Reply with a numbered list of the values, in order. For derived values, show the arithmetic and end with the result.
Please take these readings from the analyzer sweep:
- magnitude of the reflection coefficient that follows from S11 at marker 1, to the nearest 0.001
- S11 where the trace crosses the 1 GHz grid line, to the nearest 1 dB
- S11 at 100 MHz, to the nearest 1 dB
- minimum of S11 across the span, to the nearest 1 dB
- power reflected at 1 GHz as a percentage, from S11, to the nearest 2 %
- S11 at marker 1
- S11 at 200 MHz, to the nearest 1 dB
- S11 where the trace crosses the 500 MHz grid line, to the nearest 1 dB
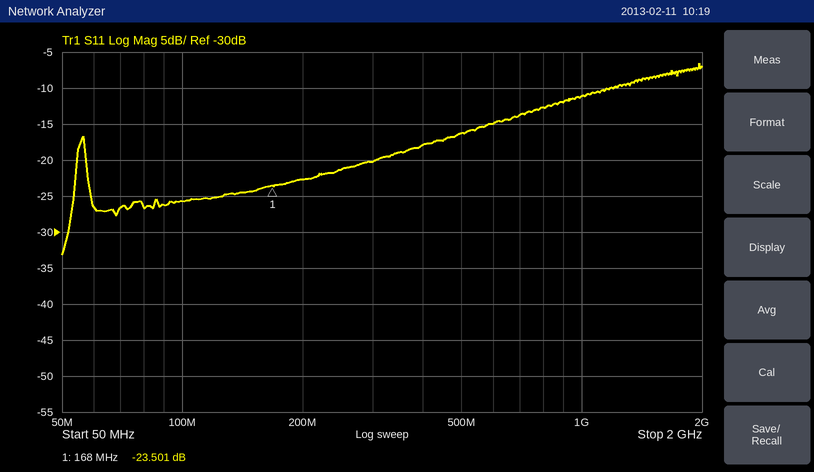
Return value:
1. 10^(-23.501/20) ≈ 0.067
2. -11 dB
3. -26 dB
4. -33 dB
5. 10^(-11/10) ≈ 8 %
6. -23.501 dB
7. -23 dB
8. -16 dB
